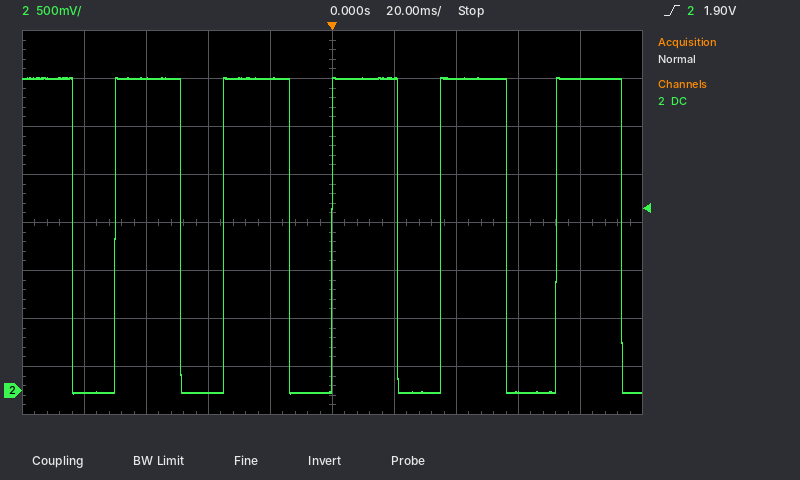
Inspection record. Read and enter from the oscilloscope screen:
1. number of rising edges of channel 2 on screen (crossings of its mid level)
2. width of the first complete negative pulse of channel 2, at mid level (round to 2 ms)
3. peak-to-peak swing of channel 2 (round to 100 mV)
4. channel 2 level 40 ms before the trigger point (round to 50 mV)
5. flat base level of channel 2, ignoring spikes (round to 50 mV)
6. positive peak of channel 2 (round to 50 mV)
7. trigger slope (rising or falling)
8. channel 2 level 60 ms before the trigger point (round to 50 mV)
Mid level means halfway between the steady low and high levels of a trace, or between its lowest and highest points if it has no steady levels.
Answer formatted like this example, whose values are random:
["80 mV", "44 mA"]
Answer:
["5", "14 ms", "3.30 V", "0 mV", "0 mV", "3.25 V", "rising", "3.25 V"]
